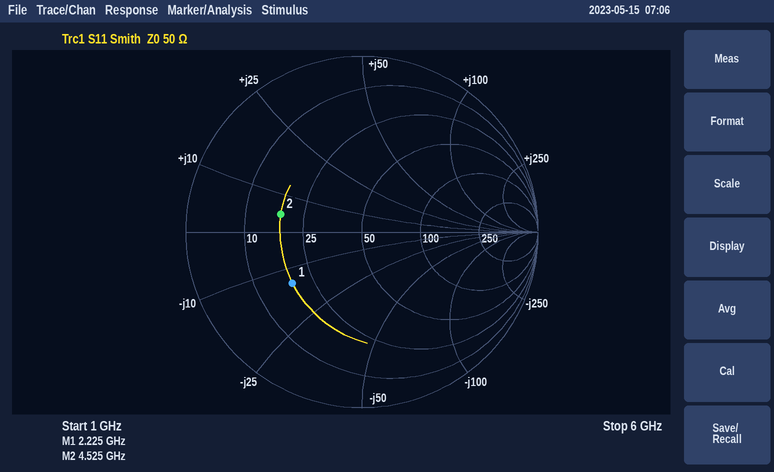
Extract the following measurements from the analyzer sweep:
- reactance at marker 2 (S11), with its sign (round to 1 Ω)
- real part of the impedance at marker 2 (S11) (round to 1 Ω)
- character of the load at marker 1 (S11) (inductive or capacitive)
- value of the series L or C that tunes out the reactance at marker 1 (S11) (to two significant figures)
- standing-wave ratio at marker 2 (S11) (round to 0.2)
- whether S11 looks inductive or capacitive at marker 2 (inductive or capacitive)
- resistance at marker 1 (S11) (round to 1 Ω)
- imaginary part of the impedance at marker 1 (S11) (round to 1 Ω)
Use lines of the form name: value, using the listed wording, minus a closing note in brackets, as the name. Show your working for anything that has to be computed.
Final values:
reactance at marker 2 (S11), with its sign: +5 Ω
real part of the impedance at marker 2 (S11): 18 Ω
character of the load at marker 1 (S11): capacitive
value of the series L or C that tunes out the reactance at marker 1 (S11): L = 14 Ω/(2π × 2.225 GHz) ≈ 1.0 nH
standing-wave ratio at marker 2 (S11): 2.8
whether S11 looks inductive or capacitive at marker 2: inductive
resistance at marker 1 (S11): 19 Ω
imaginary part of the impedance at marker 1 (S11): -14 Ω
